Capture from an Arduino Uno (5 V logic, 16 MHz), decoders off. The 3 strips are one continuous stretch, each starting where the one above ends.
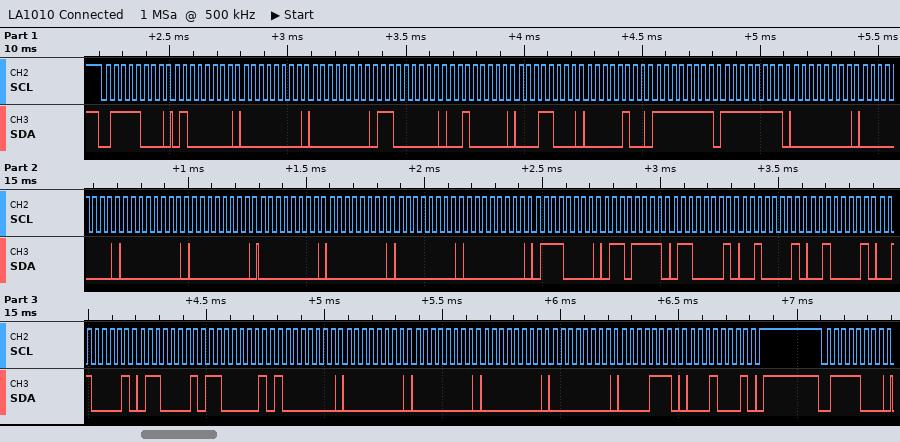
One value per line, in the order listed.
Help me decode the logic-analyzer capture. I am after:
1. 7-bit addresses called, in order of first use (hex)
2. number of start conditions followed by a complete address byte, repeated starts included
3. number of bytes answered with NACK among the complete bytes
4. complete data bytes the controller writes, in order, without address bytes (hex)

0x3C
2
0
40 00 00 C0 20 18 04 FF FF 00 00 00 00 00 00 00 00 70 6F 61 21 21 21 61 C1 80 00 00 00 00 0E 11
